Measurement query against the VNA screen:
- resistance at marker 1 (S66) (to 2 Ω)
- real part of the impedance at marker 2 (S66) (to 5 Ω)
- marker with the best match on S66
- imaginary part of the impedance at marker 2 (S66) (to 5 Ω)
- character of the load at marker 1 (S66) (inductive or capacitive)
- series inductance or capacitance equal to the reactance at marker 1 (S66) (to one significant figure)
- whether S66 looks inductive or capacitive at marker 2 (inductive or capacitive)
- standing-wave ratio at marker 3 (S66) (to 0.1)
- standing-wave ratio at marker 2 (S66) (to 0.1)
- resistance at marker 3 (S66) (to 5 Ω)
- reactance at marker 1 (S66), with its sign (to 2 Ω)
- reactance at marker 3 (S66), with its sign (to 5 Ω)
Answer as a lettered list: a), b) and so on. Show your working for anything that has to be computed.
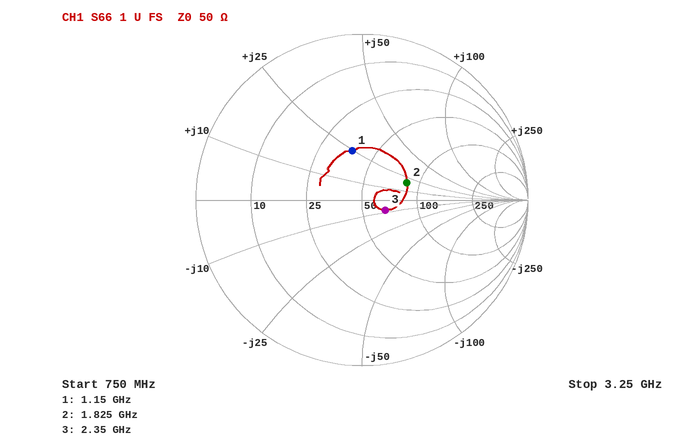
a) 38 Ω
b) 85 Ω
c) marker 3
d) +20 Ω
e) inductive
f) L = 24 Ω/(2π × 1.15 GHz) ≈ 3 nH
g) inductive
h) 1.4
i) 1.8
j) 65 Ω
k) +24 Ω
l) -10 Ω
